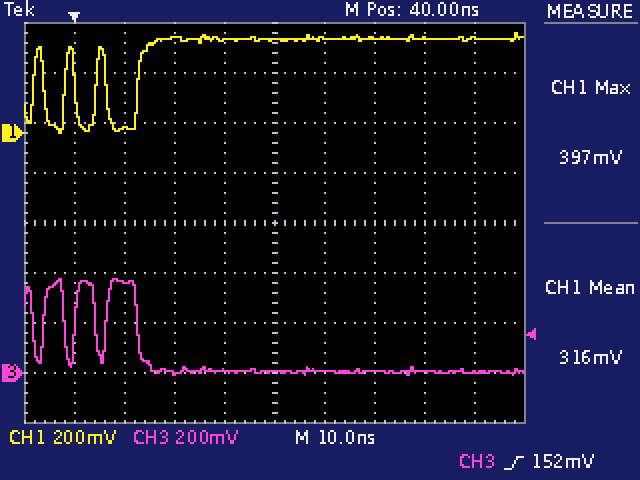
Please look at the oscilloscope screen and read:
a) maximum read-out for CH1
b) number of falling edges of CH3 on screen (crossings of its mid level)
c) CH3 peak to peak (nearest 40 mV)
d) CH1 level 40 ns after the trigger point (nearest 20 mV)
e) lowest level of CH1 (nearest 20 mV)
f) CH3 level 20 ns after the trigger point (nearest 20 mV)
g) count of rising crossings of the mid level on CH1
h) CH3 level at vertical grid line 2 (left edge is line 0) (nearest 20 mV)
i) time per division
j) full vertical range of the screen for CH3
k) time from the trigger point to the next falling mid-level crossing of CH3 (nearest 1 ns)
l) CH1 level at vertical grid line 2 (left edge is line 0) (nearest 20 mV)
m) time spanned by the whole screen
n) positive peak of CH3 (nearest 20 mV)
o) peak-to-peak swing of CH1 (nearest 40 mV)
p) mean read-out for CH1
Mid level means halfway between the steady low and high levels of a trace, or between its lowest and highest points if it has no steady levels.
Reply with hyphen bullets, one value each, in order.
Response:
- 397 mV
- 4
- 400 mV
- 380 mV
- 0 mV
- 0 mV
- 4
- 360 mV
- 10 ns
- 1.6 V
- 4 ns
- 20 mV
- 100 ns
- 380 mV
- 400 mV
- 316 mV
